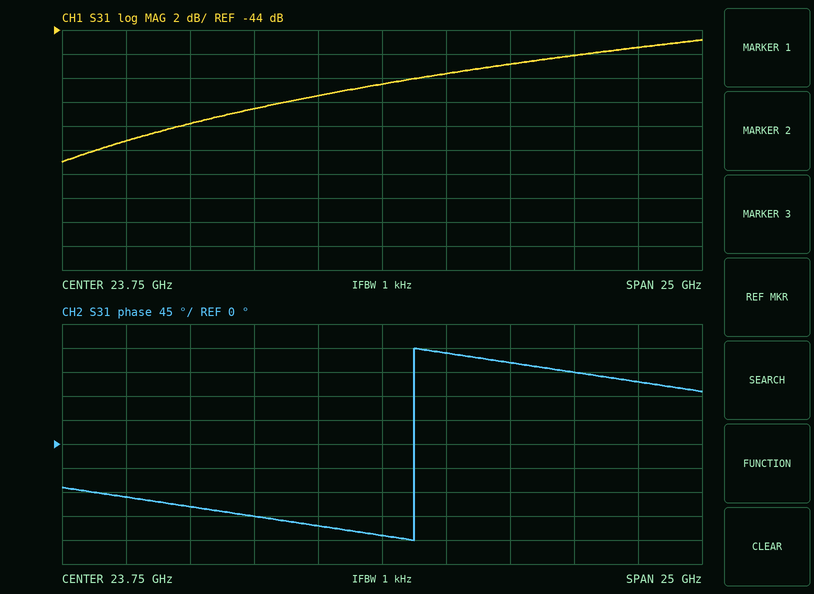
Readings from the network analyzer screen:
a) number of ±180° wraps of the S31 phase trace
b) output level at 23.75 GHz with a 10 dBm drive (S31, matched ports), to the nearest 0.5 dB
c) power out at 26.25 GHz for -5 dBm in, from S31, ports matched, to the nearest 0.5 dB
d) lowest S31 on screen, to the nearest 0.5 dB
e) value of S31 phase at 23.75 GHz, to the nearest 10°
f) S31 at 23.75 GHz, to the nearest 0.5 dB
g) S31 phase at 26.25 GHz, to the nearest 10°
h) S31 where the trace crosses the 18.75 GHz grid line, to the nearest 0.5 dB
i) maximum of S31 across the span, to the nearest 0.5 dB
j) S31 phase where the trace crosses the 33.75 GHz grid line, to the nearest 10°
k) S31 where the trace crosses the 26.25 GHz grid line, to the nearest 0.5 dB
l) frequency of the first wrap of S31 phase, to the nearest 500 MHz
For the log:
1
-38.5 dBm
-52.5 dBm
-55.0 dB
-170°
-48.5 dB
170°
-50.5 dB
-45.0 dB
120°
-47.5 dB
25.0 GHz
